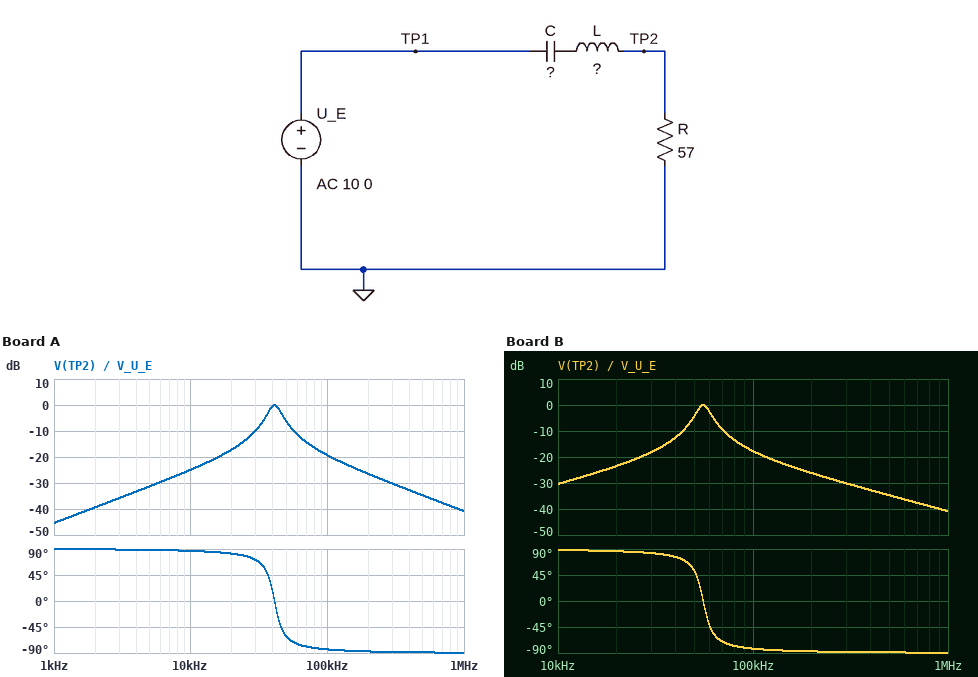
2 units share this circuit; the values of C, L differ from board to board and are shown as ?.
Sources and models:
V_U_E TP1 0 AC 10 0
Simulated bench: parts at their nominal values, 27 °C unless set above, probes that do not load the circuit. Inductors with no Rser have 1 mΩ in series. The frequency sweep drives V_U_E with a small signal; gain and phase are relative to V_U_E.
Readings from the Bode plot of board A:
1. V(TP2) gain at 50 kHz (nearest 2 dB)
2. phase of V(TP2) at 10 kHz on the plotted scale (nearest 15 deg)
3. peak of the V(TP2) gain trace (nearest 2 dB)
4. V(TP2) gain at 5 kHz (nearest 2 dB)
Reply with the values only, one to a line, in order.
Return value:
-6 dB
90 deg
0 dB
-32 dB
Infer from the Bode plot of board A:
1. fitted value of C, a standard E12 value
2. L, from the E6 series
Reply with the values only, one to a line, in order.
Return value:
15 nF
1 mH
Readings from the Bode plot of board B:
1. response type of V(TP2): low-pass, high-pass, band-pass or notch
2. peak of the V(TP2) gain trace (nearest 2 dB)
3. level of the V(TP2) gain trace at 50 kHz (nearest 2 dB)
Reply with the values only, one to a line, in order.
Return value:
band-pass
0 dB
-4 dB
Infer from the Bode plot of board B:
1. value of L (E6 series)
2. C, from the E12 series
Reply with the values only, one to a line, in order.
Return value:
1 mH
8.2 nF
